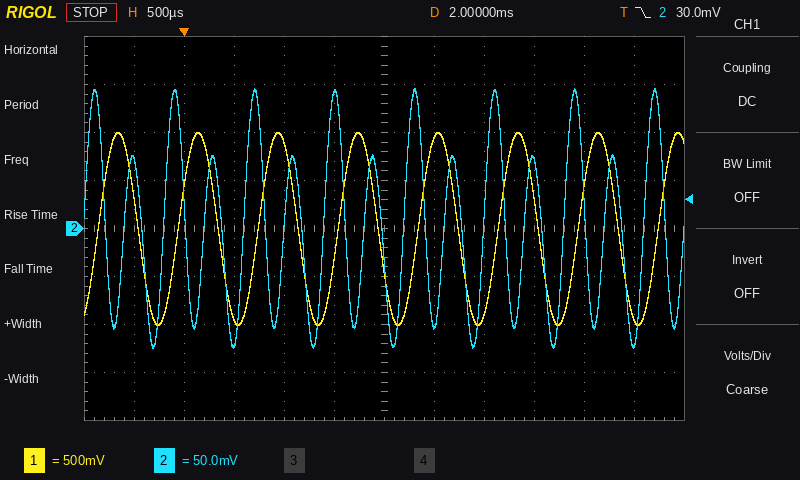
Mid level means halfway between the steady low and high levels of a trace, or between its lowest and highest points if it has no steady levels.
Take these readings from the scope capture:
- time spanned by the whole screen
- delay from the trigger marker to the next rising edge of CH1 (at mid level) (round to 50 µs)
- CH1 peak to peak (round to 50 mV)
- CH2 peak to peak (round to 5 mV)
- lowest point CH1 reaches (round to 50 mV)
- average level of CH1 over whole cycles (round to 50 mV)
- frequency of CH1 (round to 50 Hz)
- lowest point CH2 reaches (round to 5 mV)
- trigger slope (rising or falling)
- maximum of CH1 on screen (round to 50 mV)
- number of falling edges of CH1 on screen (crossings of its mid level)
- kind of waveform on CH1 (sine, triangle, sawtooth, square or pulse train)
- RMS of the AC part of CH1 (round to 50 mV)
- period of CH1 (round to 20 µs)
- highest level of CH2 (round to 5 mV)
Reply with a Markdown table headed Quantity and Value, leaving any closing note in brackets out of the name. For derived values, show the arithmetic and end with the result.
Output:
| Quantity | Value |
|---|---|
| time spanned by the whole screen | 6 ms |
| delay from the trigger marker to the next rising edge of CH1 (at mid level) | 750 µs |
| CH1 peak to peak | 1.00 V − (-1.00 V) = 2.00 V |
| CH2 peak to peak | 145 mV − (-125 mV) = 270 mV |
| lowest point CH1 reaches | -1.00 V |
| average level of CH1 over whole cycles | (1.00 V + (-1.00 V)) / 2 ≈ 0 mV |
| frequency of CH1 | 1 / 800 µs ≈ 1.25 kHz |
| lowest point CH2 reaches | -125 mV |
| trigger slope | falling |
| maximum of CH1 on screen | 1.00 V |
| number of falling edges of CH1 on screen | 7 |
| kind of waveform on CH1 | sine |
| RMS of the AC part of CH1 | 2.00 V / (2√2) ≈ 707 mV, so 700 mV to the nearest 50 mV |
| period of CH1 | 800 µs |
| highest level of CH2 | 145 mV |
